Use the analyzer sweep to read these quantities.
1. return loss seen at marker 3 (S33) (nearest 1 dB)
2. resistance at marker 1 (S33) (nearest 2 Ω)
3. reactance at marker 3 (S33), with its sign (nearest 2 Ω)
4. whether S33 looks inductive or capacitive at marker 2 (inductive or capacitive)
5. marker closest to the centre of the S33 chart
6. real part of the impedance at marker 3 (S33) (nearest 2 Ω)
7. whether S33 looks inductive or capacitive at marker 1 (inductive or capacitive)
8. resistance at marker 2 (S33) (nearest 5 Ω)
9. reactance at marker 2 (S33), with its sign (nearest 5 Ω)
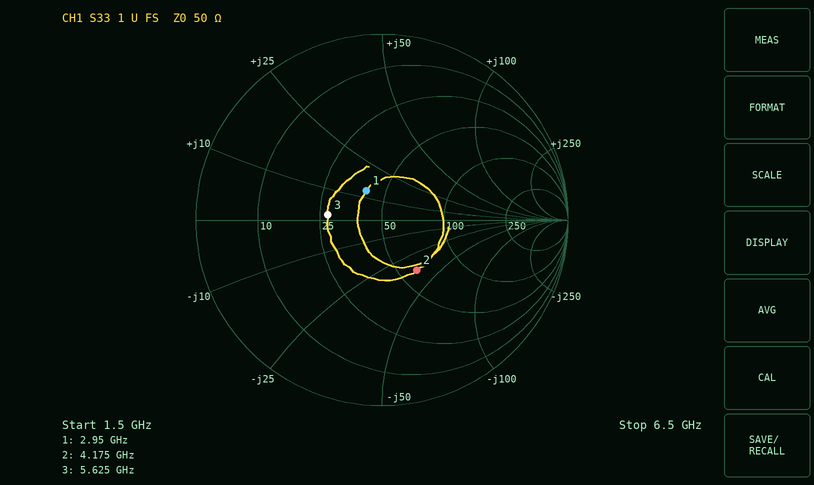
11 dB
40 Ω
+2 Ω
capacitive
marker 1
28 Ω
inductive
60 Ω
-35 Ω
